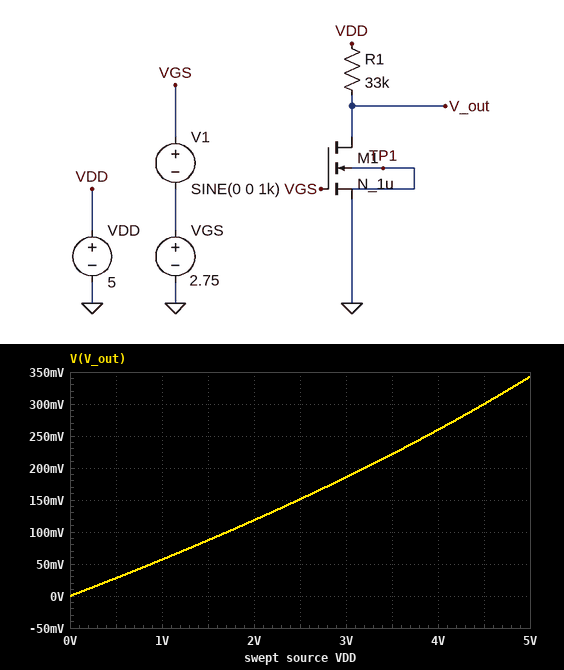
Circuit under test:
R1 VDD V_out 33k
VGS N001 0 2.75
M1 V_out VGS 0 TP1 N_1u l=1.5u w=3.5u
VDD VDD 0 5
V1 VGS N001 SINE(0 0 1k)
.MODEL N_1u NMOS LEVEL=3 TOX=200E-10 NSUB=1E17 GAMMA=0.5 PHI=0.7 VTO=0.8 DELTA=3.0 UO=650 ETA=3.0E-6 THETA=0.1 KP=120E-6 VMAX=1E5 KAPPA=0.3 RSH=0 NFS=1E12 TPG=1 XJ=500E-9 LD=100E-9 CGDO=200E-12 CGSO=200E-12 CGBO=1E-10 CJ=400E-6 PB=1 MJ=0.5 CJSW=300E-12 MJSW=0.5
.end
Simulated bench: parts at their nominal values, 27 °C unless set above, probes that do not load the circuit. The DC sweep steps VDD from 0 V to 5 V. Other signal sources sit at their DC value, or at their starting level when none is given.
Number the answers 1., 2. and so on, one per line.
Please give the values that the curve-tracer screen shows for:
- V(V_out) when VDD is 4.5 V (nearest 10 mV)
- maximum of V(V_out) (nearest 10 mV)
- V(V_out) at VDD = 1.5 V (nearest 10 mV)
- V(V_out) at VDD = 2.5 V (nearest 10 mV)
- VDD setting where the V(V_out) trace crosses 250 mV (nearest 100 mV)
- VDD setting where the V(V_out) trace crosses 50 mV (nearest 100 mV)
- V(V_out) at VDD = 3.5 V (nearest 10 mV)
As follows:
1. 300 mV
2. 340 mV
3. 90 mV
4. 150 mV
5. 3.9 V
6. 900 mV
7. 220 mV
